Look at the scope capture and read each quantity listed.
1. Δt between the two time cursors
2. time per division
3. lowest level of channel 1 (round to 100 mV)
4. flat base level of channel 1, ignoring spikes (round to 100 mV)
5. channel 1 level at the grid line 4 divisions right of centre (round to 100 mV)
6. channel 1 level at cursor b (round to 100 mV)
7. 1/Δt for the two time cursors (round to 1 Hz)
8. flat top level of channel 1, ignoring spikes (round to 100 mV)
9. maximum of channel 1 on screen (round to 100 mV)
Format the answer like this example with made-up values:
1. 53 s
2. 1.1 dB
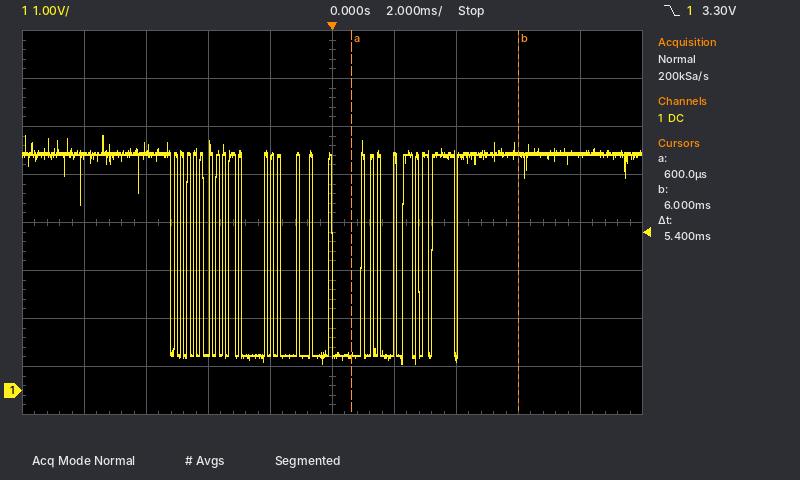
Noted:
1. 5.4 ms
2. 2 ms
3. 600 mV
4. 700 mV
5. 4.9 V
6. 4.9 V
7. 185 Hz
8. 4.9 V
9. 5.3 V
